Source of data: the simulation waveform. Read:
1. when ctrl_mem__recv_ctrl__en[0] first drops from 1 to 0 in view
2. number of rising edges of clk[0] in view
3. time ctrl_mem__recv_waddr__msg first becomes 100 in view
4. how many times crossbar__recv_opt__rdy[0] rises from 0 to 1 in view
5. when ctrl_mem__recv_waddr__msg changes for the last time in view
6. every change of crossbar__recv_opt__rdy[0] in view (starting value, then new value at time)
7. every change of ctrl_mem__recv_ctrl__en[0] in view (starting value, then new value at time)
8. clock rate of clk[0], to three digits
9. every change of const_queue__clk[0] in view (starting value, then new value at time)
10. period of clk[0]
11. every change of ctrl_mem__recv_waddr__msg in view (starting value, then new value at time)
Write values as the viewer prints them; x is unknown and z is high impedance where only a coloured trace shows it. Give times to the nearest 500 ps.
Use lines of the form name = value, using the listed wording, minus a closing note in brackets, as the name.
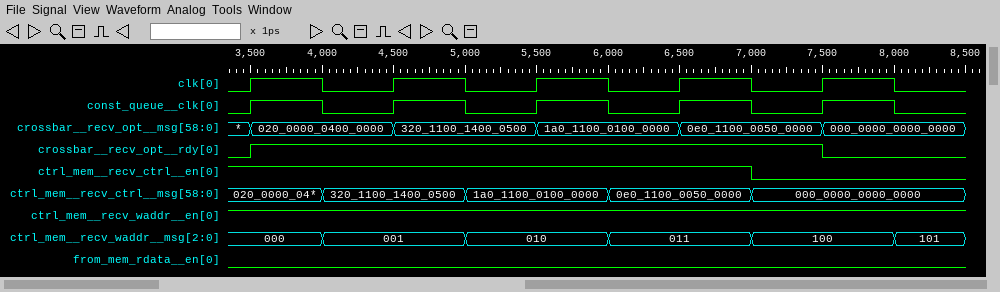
when ctrl_mem__recv_ctrl__en[0] first drops from 1 to 0 in view = 7000 ps
number of rising edges of clk[0] in view = 5
time ctrl_mem__recv_waddr__msg first becomes 100 in view = 7000 ps
how many times crossbar__recv_opt__rdy[0] rises from 0 to 1 in view = 1
when ctrl_mem__recv_waddr__msg changes for the last time in view = 8000 ps
every change of crossbar__recv_opt__rdy[0] in view = 0, 1 at 3500 ps, 0 at 7500 ps
every change of ctrl_mem__recv_ctrl__en[0] in view = 1, 0 at 7000 ps
clock rate of clk[0], to three digits = 1.00 GHz
every change of const_queue__clk[0] in view = 0, 1 at 3500 ps, 0 at 4000 ps, 1 at 4500 ps, 0 at 5000 ps, 1 at 5500 ps, 0 at 6000 ps, 1 at 6500 ps, 0 at 7000 ps, 1 at 7500 ps, 0 at 8000 ps
period of clk[0] = 1000 ps
every change of ctrl_mem__recv_waddr__msg in view = 000, 001 at 4000 ps, 010 at 5000 ps, 011 at 6000 ps, 100 at 7000 ps, 101 at 8000 ps
